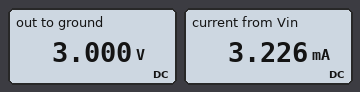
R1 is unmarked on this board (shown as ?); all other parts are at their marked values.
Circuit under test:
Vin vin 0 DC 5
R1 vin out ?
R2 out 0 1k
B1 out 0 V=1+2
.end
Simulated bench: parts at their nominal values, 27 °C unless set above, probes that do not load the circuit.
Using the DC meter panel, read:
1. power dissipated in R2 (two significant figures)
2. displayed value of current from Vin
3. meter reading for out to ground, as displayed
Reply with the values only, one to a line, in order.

9.0 mW
3.226 mA
3.000 V
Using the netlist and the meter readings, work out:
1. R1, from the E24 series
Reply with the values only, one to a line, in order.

620 Ω
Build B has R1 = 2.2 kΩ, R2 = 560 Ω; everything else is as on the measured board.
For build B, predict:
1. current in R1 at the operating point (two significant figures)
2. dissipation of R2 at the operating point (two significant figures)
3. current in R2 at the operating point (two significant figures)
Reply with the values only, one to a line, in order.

910 µA
16 mW
5.4 mA
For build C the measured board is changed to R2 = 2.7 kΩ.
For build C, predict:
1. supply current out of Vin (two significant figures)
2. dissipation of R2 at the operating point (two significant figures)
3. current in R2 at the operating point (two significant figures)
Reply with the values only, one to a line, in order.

3.2 mA
3.3 mW
1.1 mA
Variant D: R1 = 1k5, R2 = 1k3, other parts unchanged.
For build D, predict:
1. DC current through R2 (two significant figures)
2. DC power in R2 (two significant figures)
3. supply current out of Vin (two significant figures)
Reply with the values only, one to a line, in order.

2.3 mA
6.9 mW
1.3 mA
